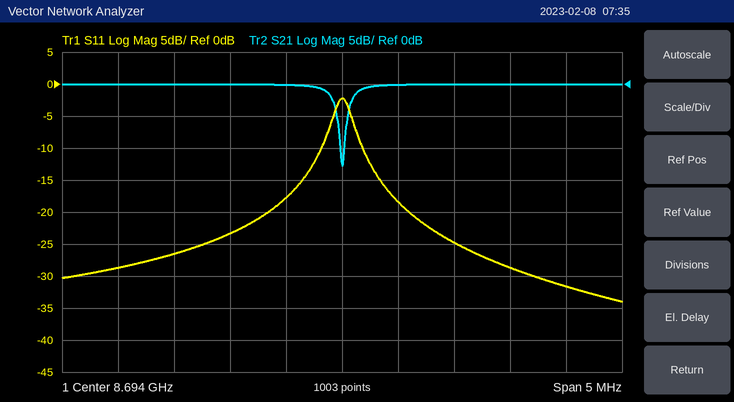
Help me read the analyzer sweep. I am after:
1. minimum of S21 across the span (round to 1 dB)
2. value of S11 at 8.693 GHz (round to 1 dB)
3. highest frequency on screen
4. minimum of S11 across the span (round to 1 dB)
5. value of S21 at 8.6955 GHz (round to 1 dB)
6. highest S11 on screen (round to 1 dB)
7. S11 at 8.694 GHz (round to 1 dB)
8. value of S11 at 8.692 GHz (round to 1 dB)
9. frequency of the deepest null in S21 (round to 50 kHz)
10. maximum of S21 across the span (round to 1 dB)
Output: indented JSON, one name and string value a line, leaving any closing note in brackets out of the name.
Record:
{
  "minimum of S21 across the span": "-13 dB",
  "value of S11 at 8.693 GHz": "-23 dB",
  "highest frequency on screen": "8.6965 GHz",
  "minimum of S11 across the span": "-34 dB",
  "value of S21 at 8.6955 GHz": "0 dB",
  "highest S11 on screen": "-2 dB",
  "S11 at 8.694 GHz": "-2 dB",
  "value of S11 at 8.692 GHz": "-29 dB",
  "frequency of the deepest null in S21": "8.69400 GHz",
  "maximum of S21 across the span": "0 dB"
}
